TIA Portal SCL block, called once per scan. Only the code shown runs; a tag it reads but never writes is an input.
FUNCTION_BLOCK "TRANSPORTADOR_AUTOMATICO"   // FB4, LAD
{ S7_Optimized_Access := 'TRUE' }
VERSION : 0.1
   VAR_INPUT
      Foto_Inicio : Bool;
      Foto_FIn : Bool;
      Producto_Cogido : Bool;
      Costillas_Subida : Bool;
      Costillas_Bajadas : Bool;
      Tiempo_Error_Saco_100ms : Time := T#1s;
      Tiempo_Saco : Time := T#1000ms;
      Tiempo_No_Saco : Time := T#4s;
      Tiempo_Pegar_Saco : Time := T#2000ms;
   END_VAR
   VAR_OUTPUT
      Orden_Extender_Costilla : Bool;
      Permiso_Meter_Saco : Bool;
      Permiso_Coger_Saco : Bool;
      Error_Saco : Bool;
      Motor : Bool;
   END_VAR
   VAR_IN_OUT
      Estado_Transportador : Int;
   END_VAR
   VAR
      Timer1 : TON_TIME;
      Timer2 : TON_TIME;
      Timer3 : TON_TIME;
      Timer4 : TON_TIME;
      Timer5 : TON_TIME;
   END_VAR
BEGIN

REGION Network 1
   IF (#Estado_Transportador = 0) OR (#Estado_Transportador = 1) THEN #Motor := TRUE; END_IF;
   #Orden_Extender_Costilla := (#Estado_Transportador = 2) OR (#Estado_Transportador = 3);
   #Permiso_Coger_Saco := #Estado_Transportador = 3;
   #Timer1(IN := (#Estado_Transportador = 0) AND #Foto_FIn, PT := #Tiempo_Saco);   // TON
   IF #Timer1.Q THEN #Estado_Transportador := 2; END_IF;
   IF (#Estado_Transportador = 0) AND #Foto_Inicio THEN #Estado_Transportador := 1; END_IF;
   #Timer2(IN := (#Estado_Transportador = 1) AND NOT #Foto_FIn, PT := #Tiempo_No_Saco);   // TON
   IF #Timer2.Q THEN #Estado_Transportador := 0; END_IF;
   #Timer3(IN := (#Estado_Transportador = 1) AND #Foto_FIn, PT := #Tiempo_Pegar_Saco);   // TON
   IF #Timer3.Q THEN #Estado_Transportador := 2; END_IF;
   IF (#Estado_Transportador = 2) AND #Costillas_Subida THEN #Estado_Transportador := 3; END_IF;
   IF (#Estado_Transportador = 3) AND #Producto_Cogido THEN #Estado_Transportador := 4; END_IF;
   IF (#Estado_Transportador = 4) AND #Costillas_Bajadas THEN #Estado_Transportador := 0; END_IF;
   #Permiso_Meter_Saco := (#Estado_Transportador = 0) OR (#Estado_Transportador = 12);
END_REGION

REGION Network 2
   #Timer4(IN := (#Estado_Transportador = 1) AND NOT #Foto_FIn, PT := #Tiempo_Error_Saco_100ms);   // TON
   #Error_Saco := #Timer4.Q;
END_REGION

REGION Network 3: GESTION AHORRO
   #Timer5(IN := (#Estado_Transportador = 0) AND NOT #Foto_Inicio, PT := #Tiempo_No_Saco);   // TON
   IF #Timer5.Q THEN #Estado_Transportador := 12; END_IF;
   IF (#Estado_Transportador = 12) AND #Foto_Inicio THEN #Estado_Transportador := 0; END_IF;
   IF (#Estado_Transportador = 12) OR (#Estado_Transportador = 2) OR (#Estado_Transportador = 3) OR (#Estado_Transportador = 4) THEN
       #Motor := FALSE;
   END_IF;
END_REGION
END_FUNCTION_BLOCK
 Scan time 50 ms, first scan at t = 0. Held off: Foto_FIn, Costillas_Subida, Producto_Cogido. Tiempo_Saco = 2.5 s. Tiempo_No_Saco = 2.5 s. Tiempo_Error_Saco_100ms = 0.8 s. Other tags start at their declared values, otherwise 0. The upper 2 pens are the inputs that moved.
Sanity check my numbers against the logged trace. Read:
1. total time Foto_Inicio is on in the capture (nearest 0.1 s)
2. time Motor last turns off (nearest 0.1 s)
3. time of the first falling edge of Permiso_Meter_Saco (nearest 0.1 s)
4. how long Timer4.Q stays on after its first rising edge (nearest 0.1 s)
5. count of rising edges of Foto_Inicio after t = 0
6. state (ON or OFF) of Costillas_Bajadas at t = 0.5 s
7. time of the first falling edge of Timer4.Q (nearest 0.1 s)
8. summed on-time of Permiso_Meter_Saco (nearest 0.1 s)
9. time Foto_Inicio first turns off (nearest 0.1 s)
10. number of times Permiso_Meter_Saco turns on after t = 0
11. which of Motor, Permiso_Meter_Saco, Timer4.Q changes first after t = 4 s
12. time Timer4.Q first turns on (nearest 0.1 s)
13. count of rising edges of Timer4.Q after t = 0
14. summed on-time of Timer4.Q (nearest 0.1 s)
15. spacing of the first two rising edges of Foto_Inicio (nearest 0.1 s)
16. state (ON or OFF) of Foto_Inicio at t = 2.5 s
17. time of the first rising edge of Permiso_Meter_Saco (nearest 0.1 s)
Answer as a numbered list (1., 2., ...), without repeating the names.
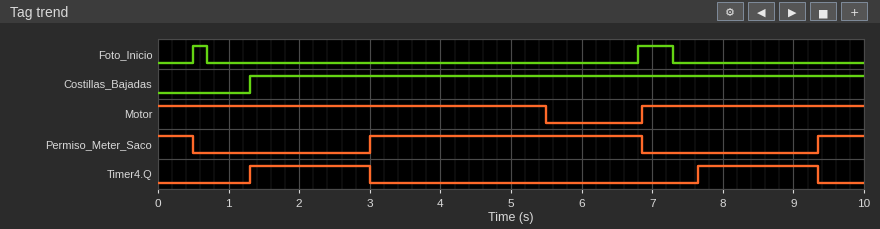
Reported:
1. 0.7 s
2. 5.5 s
3. 0.5 s
4. 1.7 s
5. 2
6. OFF
7. 3.0 s
8. 5.0 s
9. 0.7 s
10. 2
11. Motor
12. 1.3 s
13. 2
14. 3.4 s
15. 6.3 s
16. OFF
17. 3.0 s
